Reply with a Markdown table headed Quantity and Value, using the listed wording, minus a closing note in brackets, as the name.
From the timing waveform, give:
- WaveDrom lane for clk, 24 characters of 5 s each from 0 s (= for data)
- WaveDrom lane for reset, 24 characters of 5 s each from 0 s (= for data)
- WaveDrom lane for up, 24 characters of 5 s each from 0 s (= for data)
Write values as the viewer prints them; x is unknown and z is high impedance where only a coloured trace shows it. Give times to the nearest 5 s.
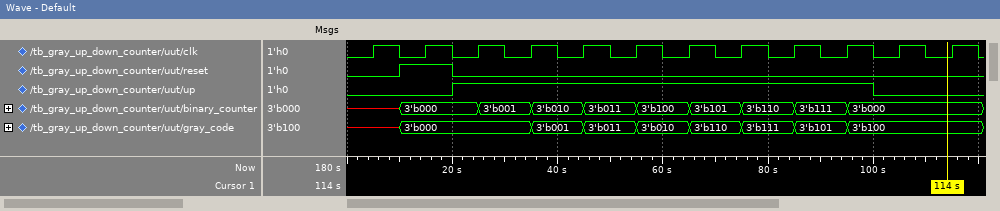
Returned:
| Quantity | Value |
|---|---|
| WaveDrom lane for clk, 24 characters of 5 s each from 0 s | {name: 'clk', wave: '010101010101010101010101'} |
| WaveDrom lane for reset, 24 characters of 5 s each from 0 s | {name: 'reset', wave: '0.1.0...................'} |
| WaveDrom lane for up, 24 characters of 5 s each from 0 s | {name: 'up', wave: '0...1...............0...'} |
